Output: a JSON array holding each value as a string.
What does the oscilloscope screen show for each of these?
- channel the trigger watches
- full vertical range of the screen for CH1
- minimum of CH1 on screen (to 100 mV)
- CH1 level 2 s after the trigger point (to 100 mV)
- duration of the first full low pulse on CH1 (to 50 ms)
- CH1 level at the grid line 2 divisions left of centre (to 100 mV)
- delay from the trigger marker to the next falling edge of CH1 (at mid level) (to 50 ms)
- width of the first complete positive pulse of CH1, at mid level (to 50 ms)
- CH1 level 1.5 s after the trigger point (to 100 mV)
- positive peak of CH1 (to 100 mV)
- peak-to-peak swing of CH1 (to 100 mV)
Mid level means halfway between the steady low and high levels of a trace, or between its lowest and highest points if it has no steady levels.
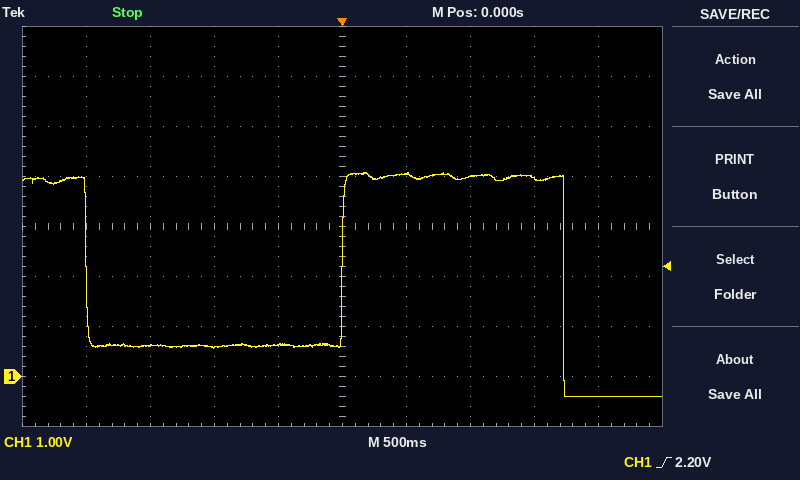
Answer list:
["CH1", "8 V", "-400 mV", "-400 mV", "2.00 s", "600 mV", "1.75 s", "1.75 s", "4.0 V", "4.1 V", "4.5 V"]
